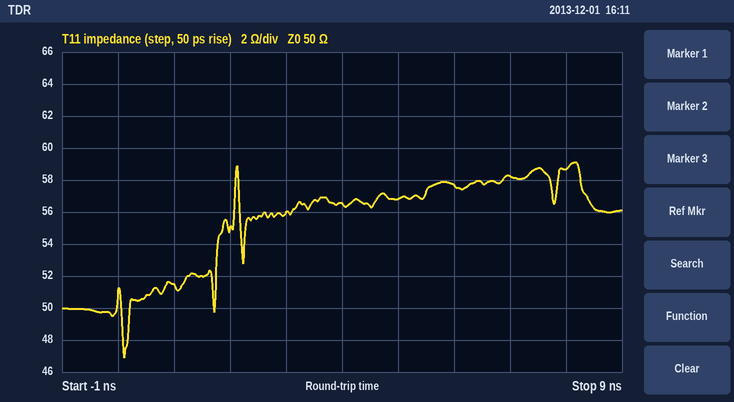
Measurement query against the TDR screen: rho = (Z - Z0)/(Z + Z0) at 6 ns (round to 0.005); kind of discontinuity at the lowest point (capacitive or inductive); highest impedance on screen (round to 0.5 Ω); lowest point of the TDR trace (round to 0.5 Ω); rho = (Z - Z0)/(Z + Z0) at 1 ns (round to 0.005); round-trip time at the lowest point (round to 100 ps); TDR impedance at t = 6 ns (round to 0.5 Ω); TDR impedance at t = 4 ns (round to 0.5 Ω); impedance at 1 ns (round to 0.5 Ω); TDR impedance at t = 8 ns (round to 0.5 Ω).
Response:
+0.070
capacitive
59.0 Ω
47.0 Ω
+0.015
100 ps
57.5 Ω
56.5 Ω
51.5 Ω
58.5 Ω
